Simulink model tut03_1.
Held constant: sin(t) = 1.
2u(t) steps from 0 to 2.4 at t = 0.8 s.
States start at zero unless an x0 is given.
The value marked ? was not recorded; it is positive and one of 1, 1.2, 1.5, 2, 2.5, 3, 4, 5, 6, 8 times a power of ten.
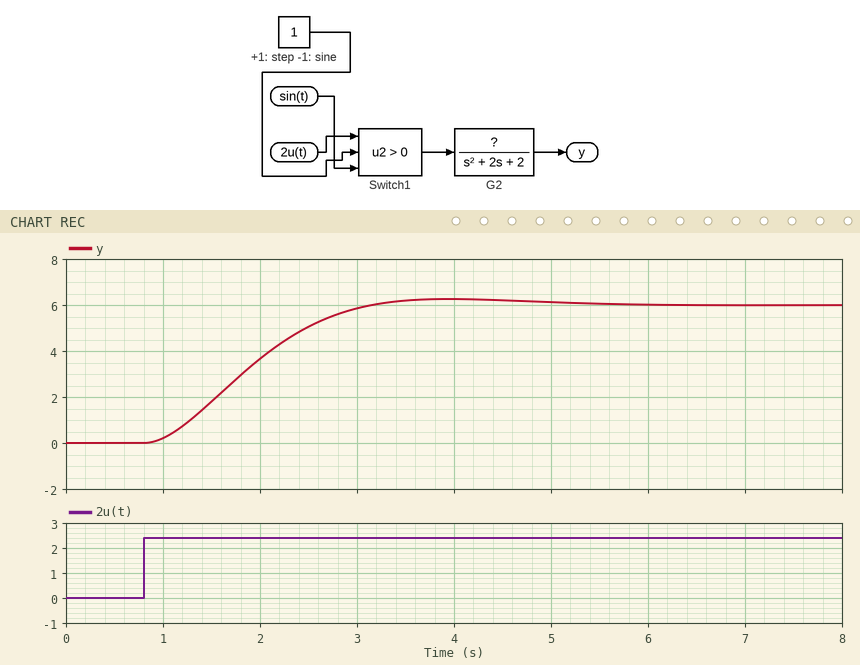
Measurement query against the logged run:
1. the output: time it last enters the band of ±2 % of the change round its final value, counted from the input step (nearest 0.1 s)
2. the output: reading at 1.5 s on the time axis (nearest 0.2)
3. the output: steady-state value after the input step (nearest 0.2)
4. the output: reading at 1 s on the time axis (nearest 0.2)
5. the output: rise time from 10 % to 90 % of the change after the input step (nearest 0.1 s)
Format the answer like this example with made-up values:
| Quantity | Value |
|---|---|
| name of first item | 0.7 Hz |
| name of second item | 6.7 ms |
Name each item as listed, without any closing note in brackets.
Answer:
| Quantity | Value |
|---|---|
| the output: time it last enters the band of ±2 % of the change round its final value, counted from the input step | 4.2 s |
| the output: reading at 1.5 s on the time axis | 1.8 |
| the output: steady-state value after the input step | 6.0 |
| the output: reading at 1 s on the time axis | 0.2 |
| the output: rise time from 10 % to 90 % of the change after the input step | 1.5 s |
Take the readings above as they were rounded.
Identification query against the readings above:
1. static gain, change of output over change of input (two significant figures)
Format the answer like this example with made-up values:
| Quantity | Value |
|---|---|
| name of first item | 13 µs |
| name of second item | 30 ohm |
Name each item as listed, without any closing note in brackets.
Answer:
| Quantity | Value |
|---|---|
| static gain, change of output over change of input | 2.5 |
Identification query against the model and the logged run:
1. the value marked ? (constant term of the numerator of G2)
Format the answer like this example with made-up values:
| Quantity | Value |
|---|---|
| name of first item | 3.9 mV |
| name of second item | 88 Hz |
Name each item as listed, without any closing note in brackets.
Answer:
| Quantity | Value |
|---|---|
| the value marked ? | 5 |
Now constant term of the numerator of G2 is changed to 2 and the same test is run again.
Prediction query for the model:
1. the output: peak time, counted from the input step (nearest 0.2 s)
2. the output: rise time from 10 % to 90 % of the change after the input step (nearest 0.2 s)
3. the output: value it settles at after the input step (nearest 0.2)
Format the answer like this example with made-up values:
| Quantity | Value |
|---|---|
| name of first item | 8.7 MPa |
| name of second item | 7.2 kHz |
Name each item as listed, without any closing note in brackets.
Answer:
| Quantity | Value |
|---|---|
| the output: peak time, counted from the input step | 3.2 s |
| the output: rise time from 10 % to 90 % of the change after the input step | 1.6 s |
| the output: value it settles at after the input step | 2.4 |
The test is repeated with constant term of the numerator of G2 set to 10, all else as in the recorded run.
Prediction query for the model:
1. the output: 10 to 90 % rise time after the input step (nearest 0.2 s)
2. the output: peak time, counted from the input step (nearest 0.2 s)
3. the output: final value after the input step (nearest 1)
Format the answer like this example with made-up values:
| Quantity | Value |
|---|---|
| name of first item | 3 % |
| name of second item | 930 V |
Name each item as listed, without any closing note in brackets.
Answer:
| Quantity | Value |
|---|---|
| the output: 10 to 90 % rise time after the input step | 1.6 s |
| the output: peak time, counted from the input step | 3.2 s |
| the output: final value after the input step | 12 |
